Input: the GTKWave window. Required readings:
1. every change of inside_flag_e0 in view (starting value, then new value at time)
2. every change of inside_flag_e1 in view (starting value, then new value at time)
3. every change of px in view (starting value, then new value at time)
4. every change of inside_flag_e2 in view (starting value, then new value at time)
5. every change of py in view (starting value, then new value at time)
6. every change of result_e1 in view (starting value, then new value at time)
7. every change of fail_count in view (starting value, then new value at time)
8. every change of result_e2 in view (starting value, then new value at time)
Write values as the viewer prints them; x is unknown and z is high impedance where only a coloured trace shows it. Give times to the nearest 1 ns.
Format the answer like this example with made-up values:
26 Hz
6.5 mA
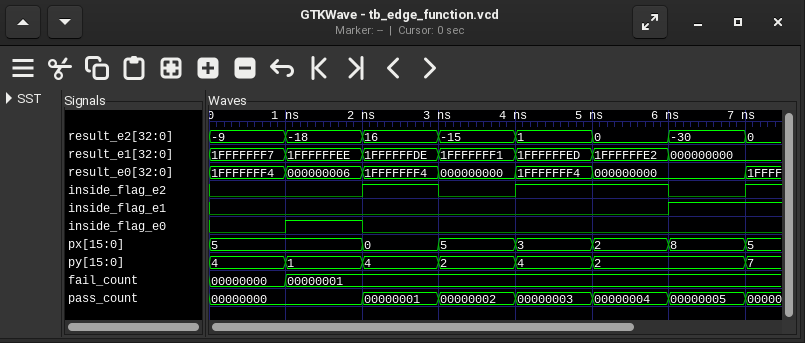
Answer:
0, 1 at 1 ns, 0 at 2 ns
0, 1 at 6 ns
5, 0 at 2 ns, 5 at 3 ns, 3 at 4 ns, 2 at 5 ns, 8 at 6 ns, 5 at 7 ns
0, 1 at 2 ns, 0 at 3 ns, 1 at 4 ns, 0 at 6 ns, 1 at 7 ns
4, 1 at 1 ns, 4 at 2 ns, 2 at 3 ns, 4 at 4 ns, 2 at 5 ns, 7 at 7 ns
1FFFFFFF7, 1FFFFFFEE at 1 ns, 1FFFFFFDE at 2 ns, 1FFFFFFF1 at 3 ns, 1FFFFFFED at 4 ns, 1FFFFFFE2 at 5 ns, 000000000 at 6 ns
00000000, 00000001 at 1 ns
-9, -18 at 1 ns, 16 at 2 ns, -15 at 3 ns, 1 at 4 ns, 0 at 5 ns, -30 at 6 ns, 0 at 7 ns
